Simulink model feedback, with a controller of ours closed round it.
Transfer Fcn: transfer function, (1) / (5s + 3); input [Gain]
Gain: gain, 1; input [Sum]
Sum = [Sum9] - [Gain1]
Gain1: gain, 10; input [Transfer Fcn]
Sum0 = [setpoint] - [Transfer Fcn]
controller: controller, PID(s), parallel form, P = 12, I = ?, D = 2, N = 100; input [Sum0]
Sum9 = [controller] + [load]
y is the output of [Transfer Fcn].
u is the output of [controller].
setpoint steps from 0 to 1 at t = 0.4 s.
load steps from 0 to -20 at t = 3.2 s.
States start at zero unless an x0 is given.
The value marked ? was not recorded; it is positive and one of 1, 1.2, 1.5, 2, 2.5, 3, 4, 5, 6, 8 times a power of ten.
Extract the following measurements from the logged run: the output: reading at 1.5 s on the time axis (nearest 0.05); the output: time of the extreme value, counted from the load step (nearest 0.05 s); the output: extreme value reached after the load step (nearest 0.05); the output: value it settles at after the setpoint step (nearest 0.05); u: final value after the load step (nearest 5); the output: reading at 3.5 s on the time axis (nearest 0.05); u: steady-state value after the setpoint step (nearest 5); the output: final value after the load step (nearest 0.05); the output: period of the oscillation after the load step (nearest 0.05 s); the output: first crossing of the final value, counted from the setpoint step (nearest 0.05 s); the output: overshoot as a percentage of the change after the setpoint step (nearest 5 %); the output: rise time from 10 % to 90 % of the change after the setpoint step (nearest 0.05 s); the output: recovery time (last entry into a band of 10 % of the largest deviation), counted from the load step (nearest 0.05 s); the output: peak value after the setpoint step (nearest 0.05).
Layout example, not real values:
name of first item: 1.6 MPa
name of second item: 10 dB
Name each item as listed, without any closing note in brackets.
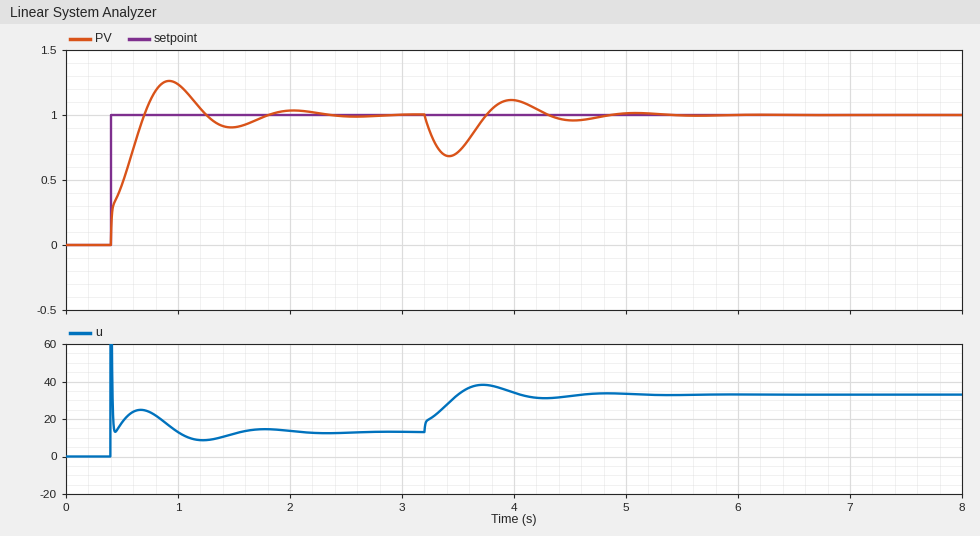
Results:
the output: reading at 1.5 s on the time axis: 0.90
the output: time of the extreme value, counted from the load step: 0.20 s
the output: extreme value reached after the load step: 0.70
the output: value it settles at after the setpoint step: 1.00
u: final value after the load step: 35
the output: reading at 3.5 s on the time axis: 0.70
u: steady-state value after the setpoint step: 15
the output: final value after the load step: 1.00
the output: period of the oscillation after the load step: 1.10 s
the output: first crossing of the final value, counted from the setpoint step: 0.30 s
the output: overshoot as a percentage of the change after the setpoint step: 25 %
the output: rise time from 10 % to 90 % of the change after the setpoint step: 0.25 s
the output: recovery time (last entry into a band of 10 % of the largest deviation), counted from the load step: 1.45 s
the output: peak value after the setpoint step: 1.25
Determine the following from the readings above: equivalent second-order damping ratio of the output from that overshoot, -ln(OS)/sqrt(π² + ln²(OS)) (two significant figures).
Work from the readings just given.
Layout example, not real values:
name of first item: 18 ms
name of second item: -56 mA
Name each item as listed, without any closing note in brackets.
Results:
equivalent second-order damping ratio of the output from that overshoot, -ln(OS)/sqrt(π² + ln²(OS)): 0.40
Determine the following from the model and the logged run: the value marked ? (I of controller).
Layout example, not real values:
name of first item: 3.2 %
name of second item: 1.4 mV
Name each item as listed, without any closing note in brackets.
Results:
the value marked ?: 250
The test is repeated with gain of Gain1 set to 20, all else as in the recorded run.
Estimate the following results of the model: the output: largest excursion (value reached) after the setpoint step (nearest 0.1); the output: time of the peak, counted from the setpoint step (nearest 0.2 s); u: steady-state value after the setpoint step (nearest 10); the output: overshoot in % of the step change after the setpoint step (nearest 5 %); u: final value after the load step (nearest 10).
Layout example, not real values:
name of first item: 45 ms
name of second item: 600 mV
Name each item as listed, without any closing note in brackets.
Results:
the output: largest excursion (value reached) after the setpoint step: 1.2
the output: time of the peak, counted from the setpoint step: 0.6 s
u: steady-state value after the setpoint step: 20
the output: overshoot in % of the step change after the setpoint step: 15 %
u: final value after the load step: 40
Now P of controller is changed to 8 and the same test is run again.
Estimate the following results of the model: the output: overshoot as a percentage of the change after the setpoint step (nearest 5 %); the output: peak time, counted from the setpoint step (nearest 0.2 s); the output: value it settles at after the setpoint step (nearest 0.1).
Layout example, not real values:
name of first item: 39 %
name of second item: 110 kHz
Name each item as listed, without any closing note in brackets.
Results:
the output: overshoot as a percentage of the change after the setpoint step: 30 %
the output: peak time, counted from the setpoint step: 0.6 s
the output: value it settles at after the setpoint step: 1.0
